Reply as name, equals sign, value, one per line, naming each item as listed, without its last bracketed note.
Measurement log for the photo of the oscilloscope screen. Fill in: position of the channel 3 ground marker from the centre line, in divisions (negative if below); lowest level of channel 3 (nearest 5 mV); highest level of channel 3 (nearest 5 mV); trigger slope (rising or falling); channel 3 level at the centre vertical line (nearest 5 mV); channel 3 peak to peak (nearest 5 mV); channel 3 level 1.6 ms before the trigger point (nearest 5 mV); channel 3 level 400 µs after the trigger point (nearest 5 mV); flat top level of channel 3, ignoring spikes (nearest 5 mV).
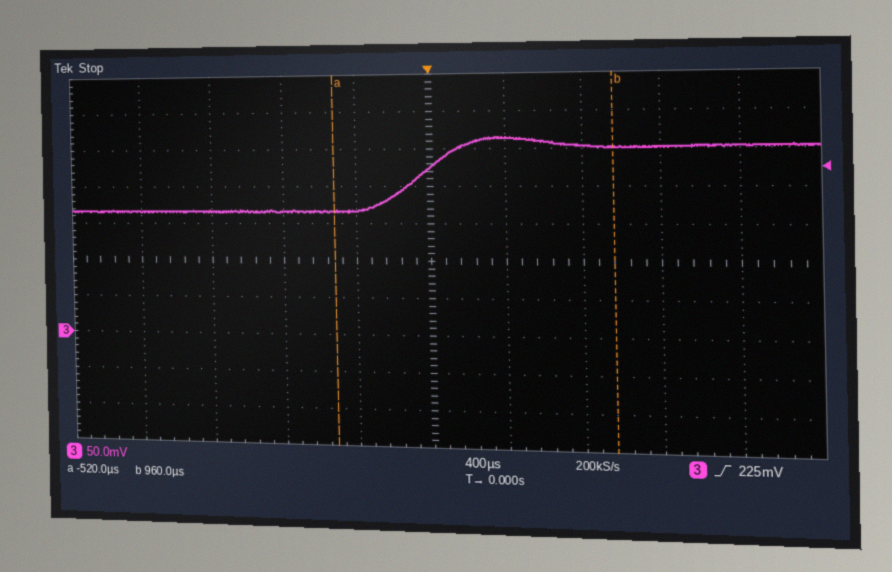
position of the channel 3 ground marker from the centre line, in divisions = -2.0 div
lowest level of channel 3 = 165 mV
highest level of channel 3 = 265 mV
trigger slope = rising
channel 3 level at the centre vertical line = 225 mV
channel 3 peak to peak = 100 mV
channel 3 level 1.6 ms before the trigger point = 165 mV
channel 3 level 400 µs after the trigger point = 265 mV
flat top level of channel 3, ignoring spikes = 255 mV
